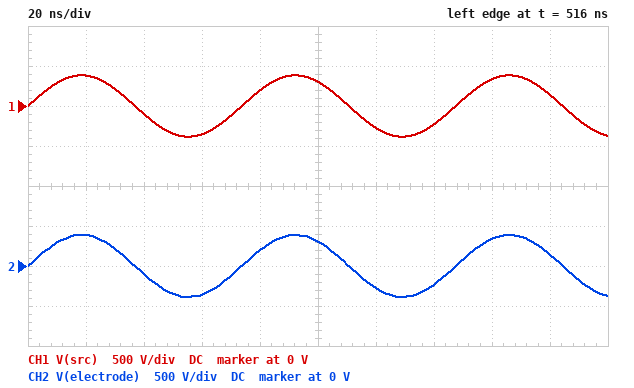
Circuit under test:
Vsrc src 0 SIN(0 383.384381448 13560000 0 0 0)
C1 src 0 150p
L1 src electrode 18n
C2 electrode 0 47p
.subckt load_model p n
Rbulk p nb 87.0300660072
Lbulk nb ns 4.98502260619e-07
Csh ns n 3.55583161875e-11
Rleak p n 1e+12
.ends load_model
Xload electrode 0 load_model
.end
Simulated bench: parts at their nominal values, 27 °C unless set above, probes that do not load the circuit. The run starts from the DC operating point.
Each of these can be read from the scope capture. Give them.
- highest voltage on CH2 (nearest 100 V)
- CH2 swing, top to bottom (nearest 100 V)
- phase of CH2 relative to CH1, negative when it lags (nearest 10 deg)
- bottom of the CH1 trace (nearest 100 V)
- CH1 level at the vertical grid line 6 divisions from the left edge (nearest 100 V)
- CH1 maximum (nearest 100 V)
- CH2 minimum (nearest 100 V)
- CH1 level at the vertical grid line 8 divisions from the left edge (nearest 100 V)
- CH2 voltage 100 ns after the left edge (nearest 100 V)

400 V
800 V
0 deg
-400 V
-300 V
400 V
-400 V
300 V
300 V
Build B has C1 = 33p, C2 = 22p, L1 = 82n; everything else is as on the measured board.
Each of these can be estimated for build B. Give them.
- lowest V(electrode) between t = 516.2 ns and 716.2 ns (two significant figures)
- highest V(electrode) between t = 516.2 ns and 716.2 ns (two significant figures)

-400 V
400 V
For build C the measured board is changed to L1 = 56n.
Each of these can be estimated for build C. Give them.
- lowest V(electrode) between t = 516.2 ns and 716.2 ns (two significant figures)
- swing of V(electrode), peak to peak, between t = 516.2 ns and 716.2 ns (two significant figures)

-400 V
790 V
